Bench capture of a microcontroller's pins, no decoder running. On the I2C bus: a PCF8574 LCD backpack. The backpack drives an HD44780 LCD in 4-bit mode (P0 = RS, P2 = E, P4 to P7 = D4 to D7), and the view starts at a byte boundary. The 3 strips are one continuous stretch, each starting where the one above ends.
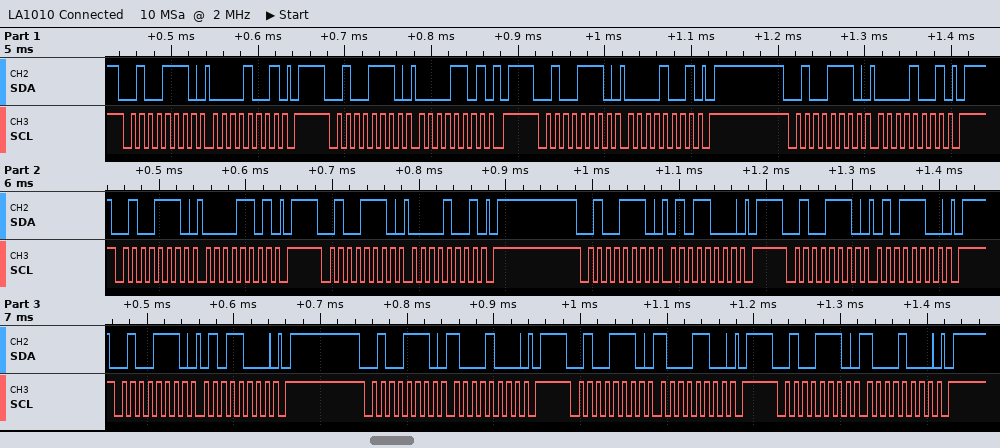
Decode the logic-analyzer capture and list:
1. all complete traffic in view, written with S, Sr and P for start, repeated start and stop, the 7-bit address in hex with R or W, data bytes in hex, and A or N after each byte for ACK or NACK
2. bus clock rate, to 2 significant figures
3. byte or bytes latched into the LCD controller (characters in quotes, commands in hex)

S 27W A 09 A P S 27W A 0D A P S 27W A 09 A P S 27W A 09 A P S 27W A 0D A P S 27W A 09 A P S 27W A 58 A P S 27W A 5C A P S 27W A 58 A P S 27W A 88 A P S 27W A 8C A P S 27W A 88 A P
100 kHz
data 0x00 0x58
